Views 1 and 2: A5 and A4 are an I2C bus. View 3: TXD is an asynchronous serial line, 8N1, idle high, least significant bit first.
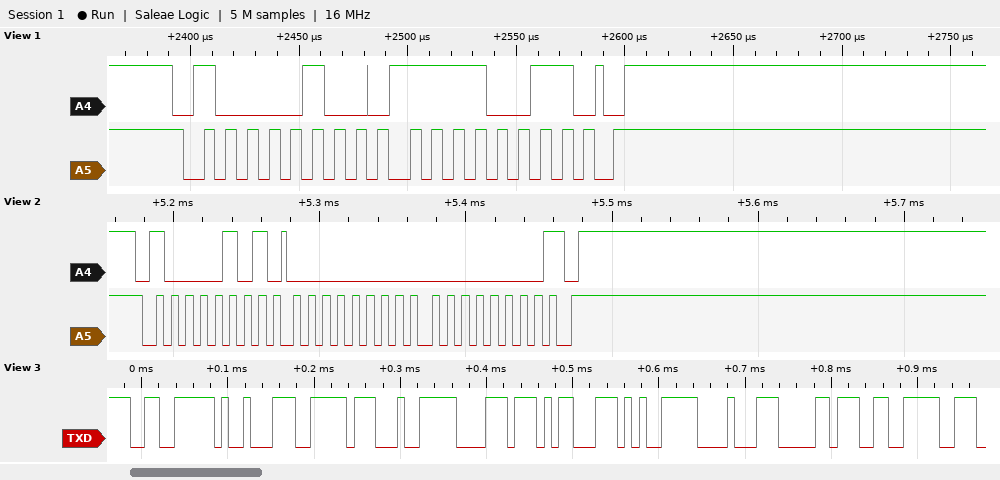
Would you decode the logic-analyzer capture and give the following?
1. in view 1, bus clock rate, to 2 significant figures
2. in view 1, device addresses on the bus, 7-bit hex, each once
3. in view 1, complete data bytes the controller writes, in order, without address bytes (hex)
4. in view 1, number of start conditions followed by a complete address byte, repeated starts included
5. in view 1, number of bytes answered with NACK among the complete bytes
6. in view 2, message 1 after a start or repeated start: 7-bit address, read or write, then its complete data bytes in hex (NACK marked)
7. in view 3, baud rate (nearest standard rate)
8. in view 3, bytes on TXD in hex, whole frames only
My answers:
100 kHz
0x42
F3
1
0
0x42 read: 00 00 NACK
115200 baud
E6 89 BE E4 B8 8D E5 88 B0 E6
